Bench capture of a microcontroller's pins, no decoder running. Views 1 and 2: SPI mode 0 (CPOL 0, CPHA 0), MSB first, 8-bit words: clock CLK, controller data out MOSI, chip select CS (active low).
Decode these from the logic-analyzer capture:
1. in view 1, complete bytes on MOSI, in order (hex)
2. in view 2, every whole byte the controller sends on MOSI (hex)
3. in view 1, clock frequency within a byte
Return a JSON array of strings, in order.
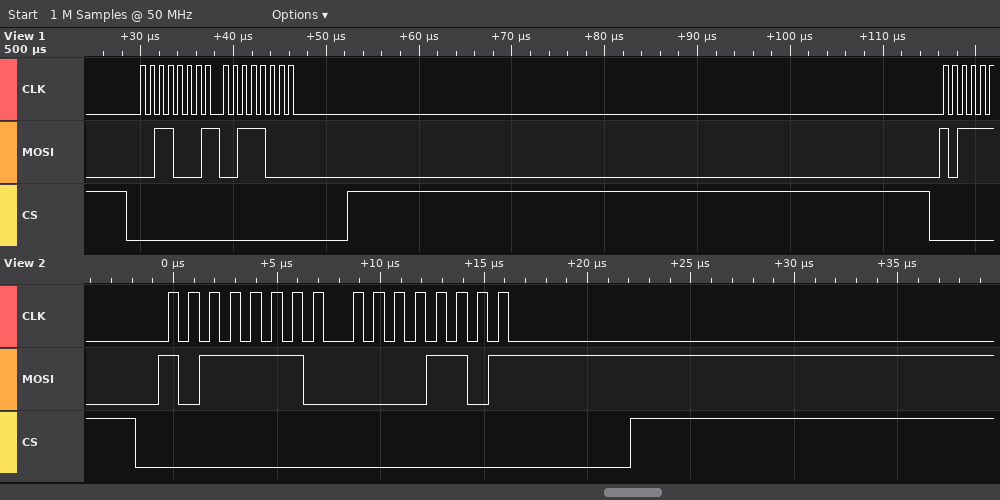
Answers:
["0x31 0x38", "0xBE 0x0D", "1 MHz"]
